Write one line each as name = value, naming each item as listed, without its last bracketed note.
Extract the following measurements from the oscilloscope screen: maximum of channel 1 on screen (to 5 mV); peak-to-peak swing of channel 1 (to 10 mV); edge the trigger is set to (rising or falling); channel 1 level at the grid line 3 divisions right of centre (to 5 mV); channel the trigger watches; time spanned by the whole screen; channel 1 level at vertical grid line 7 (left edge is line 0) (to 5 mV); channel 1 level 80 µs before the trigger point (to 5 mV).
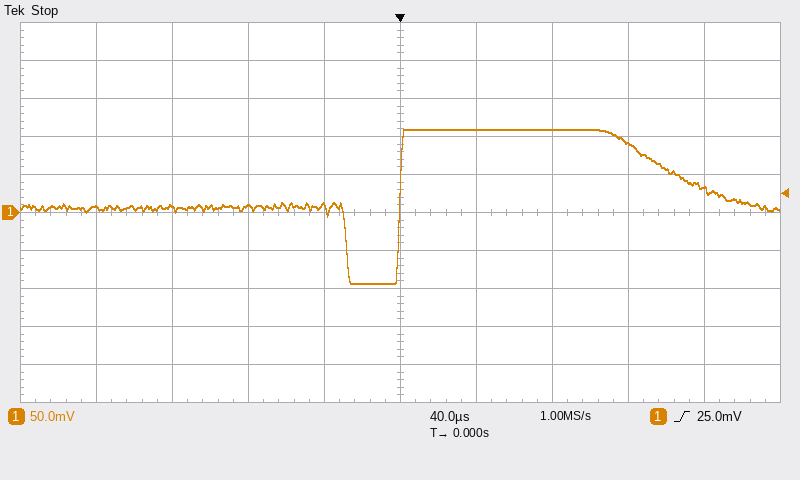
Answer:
maximum of channel 1 on screen = 110 mV
peak-to-peak swing of channel 1 = 200 mV
edge the trigger is set to = rising
channel 1 level at the grid line 3 divisions right of centre = 90 mV
channel the trigger watches = channel 1
time spanned by the whole screen = 400 µs
channel 1 level at vertical grid line 7 (left edge is line 0) = 110 mV
channel 1 level 80 µs before the trigger point = 10 mV
